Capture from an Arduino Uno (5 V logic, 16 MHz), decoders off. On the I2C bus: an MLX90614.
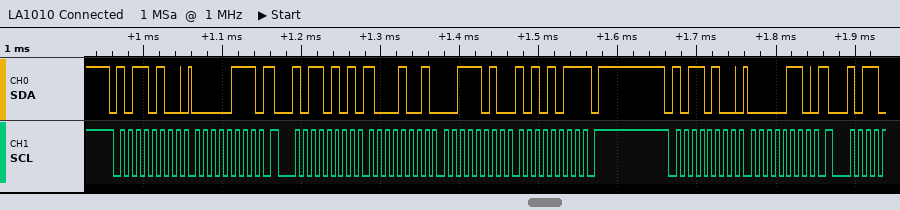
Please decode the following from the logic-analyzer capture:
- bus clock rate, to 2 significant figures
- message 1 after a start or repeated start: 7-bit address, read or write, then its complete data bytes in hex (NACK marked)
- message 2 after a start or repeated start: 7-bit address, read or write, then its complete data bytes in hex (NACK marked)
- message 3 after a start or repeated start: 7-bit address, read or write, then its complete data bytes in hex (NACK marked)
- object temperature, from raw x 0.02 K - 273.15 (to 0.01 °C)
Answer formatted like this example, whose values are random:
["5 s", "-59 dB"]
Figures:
["100 kHz", "0x5A write: 07", "0x5A read: 89 3A AB NACK", "0x5A write: 06", "26.55 °C"]
